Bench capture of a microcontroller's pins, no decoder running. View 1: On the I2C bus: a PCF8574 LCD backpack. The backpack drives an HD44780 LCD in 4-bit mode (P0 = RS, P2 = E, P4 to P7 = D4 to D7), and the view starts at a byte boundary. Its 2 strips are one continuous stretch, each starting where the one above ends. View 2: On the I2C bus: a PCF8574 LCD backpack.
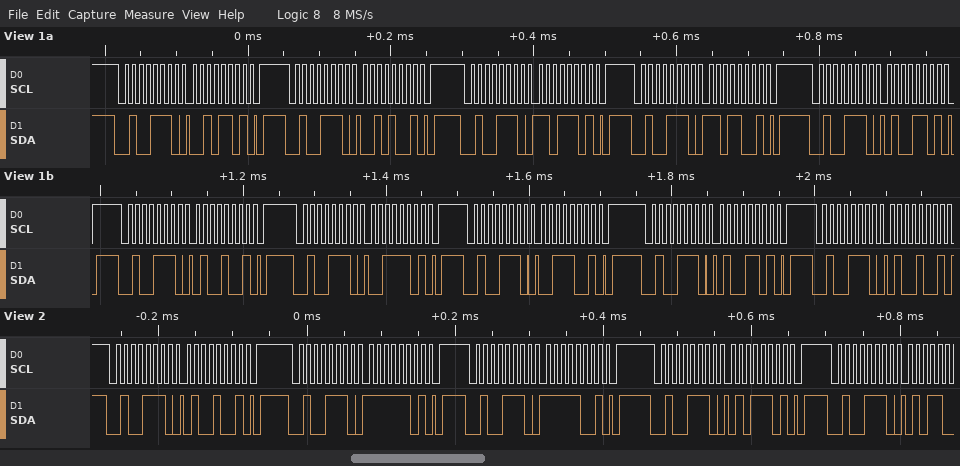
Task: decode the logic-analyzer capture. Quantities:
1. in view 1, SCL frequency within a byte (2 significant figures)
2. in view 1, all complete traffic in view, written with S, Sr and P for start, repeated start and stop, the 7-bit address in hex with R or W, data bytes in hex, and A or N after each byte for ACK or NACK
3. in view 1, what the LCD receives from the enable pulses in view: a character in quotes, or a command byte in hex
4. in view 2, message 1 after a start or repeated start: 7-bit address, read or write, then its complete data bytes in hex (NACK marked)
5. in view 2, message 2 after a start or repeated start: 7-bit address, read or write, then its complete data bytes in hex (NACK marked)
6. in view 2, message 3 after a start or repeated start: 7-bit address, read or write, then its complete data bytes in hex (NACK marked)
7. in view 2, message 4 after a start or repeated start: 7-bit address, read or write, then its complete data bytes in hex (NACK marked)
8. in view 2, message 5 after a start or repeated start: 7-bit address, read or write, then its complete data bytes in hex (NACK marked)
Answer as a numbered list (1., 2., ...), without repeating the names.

1. 100 kHz
2. S 27W A 2D A P S 27W A 29 A P S 27W A DD A P S 27W A D9 A P S 27W A 4D A P S 27W A 49 A P S 27W A 3D A P S 27W A 39 A P S 27W A 4D A P S 27W A 49 A
3. '-' 'C'
4. 0x27 write: 49
5. 0x27 write: FD
6. 0x27 write: F9
7. 0x27 write: 5D
8. 0x27 write
